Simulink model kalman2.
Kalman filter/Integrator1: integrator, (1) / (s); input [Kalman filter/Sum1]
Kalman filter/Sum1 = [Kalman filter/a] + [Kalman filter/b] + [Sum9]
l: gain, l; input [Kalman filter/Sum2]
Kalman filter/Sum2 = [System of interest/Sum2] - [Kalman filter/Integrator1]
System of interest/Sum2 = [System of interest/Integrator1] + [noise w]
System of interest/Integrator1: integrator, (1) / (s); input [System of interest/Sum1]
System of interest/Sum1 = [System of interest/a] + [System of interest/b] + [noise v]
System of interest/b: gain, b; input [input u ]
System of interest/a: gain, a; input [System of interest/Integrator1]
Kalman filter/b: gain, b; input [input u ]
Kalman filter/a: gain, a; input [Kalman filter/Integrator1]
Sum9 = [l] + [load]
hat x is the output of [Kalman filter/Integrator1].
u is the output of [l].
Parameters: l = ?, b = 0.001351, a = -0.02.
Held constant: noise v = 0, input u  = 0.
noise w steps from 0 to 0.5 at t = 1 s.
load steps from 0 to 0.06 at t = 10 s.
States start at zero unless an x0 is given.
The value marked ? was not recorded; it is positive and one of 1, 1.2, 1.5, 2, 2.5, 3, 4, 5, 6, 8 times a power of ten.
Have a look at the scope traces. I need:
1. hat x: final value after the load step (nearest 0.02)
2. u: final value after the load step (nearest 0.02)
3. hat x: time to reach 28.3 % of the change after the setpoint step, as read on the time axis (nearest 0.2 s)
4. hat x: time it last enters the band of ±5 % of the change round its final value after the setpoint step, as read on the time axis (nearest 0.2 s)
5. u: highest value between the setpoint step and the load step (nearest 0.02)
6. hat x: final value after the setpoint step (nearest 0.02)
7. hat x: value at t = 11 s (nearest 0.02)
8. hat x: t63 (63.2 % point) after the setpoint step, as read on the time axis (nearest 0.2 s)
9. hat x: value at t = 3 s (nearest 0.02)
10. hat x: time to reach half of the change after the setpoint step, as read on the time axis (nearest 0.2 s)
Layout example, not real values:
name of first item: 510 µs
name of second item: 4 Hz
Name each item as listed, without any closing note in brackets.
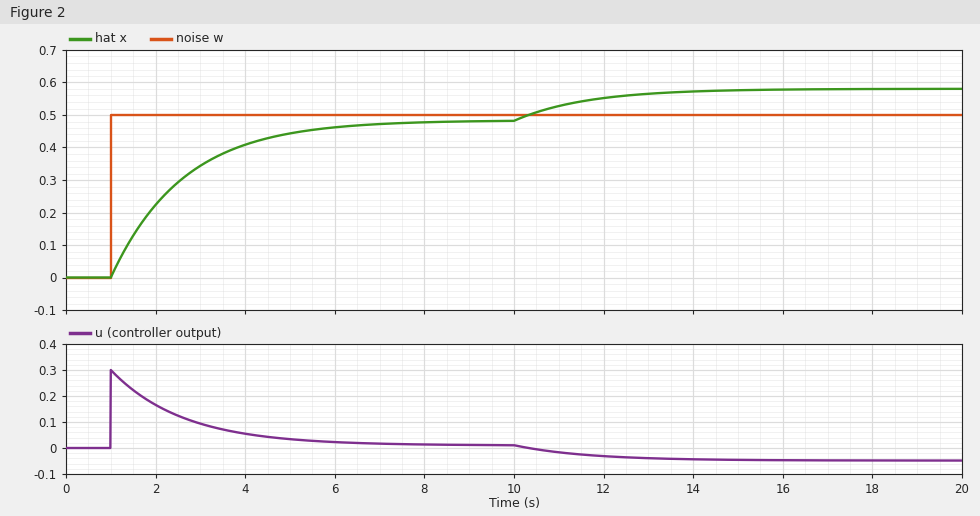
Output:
hat x: final value after the load step: 0.58
u: final value after the load step: -0.04
hat x: time to reach 28.3 % of the change after the setpoint step, as read on the time axis: 1.6 s
hat x: time it last enters the band of ±5 % of the change round its final value after the setpoint step, as read on the time axis: 5.8 s
u: highest value between the setpoint step and the load step: 0.30
hat x: final value after the setpoint step: 0.48
hat x: value at t = 11 s: 0.52
hat x: t63 (63.2 % point) after the setpoint step, as read on the time axis: 2.6 s
hat x: value at t = 3 s: 0.34
hat x: time to reach half of the change after the setpoint step, as read on the time axis: 2.2 s
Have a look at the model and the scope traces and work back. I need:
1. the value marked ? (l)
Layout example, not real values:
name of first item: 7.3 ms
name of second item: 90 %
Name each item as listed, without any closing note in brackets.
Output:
the value marked ?: 0.6
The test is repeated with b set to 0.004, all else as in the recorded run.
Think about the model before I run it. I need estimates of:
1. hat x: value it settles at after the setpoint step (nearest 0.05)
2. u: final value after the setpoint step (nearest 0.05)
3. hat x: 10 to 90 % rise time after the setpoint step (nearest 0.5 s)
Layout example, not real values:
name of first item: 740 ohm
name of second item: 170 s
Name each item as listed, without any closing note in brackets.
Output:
hat x: value it settles at after the setpoint step: 0.50
u: final value after the setpoint step: 0.00
hat x: 10 to 90 % rise time after the setpoint step: 3.5 s
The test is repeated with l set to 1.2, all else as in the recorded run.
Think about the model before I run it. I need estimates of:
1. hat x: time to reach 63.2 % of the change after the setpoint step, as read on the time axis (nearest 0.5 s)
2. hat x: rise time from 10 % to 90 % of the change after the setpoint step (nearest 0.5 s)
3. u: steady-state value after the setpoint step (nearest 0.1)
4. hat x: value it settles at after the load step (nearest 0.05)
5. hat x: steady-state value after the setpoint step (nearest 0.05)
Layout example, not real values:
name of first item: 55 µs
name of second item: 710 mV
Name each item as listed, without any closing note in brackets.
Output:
hat x: time to reach 63.2 % of the change after the setpoint step, as read on the time axis: 2.0 s
hat x: rise time from 10 % to 90 % of the change after the setpoint step: 2.0 s
u: steady-state value after the setpoint step: 0.0
hat x: value it settles at after the load step: 0.55
hat x: steady-state value after the setpoint step: 0.50
